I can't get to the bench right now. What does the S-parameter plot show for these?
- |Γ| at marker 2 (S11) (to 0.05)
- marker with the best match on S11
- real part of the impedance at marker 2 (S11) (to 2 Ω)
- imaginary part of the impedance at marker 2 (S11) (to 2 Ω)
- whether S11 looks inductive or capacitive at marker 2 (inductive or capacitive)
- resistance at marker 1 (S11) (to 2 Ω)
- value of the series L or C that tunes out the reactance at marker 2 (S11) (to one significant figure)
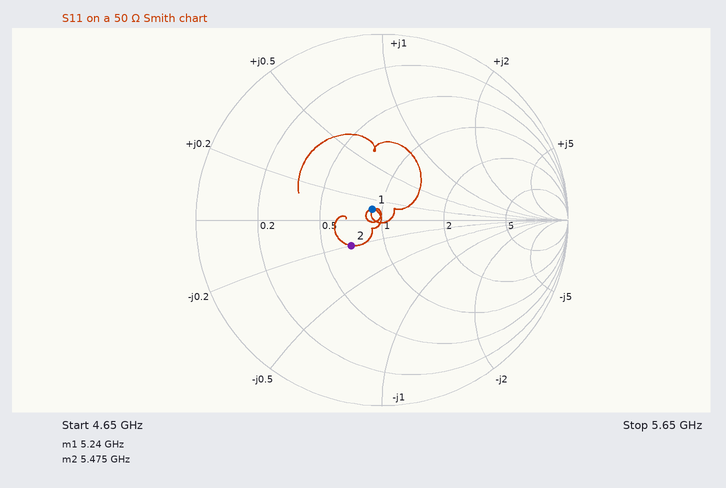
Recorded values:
0.20
marker 1
34 Ω
-10 Ω
capacitive
44 Ω
300 pH
